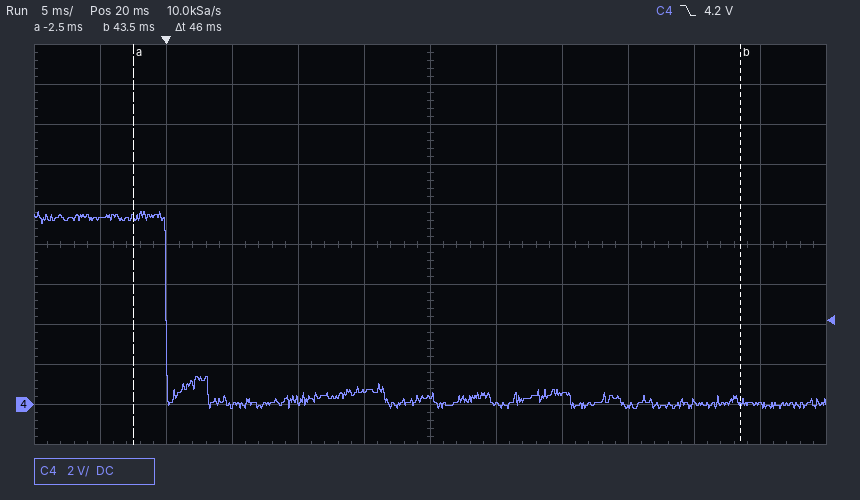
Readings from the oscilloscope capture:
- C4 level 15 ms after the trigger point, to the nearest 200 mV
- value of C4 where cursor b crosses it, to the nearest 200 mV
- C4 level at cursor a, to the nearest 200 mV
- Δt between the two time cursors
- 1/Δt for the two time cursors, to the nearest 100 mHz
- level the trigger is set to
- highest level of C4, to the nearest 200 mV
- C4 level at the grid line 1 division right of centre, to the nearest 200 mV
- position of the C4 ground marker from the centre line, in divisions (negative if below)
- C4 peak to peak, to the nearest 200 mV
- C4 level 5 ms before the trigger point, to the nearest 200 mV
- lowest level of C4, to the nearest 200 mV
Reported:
600 mV
200 mV
9.4 V
46 ms
21.7 Hz
4.2 V
9.6 V
0.0 V
-4.0 div
9.8 V
9.2 V
-200 mV
